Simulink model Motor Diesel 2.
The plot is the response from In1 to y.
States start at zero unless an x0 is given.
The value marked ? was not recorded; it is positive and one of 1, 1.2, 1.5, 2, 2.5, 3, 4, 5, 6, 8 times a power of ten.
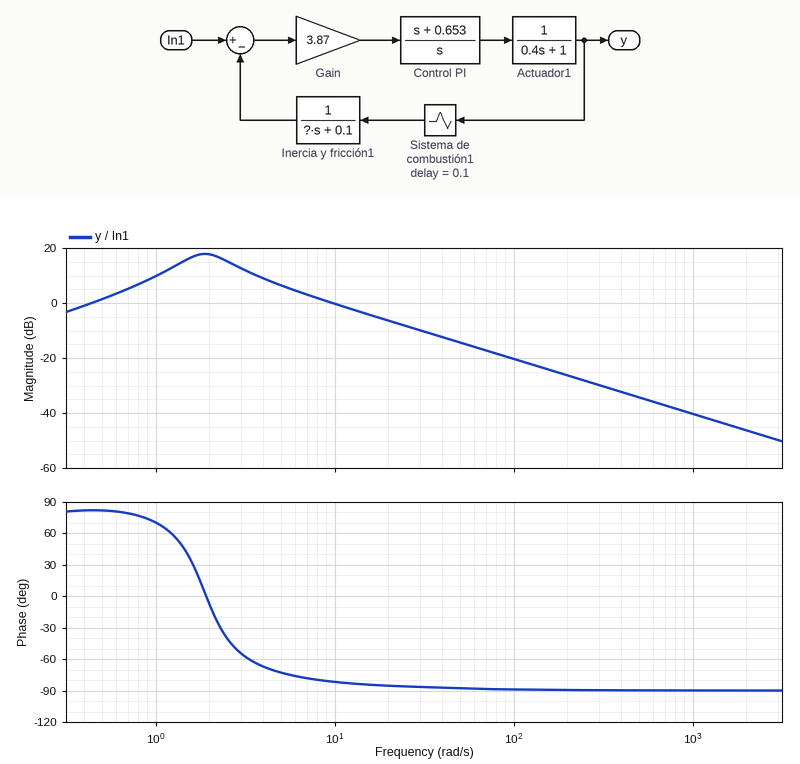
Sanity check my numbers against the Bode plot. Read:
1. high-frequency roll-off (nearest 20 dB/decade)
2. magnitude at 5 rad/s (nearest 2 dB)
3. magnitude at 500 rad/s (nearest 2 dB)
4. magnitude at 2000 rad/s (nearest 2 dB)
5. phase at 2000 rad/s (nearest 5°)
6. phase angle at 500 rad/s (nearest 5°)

-20 dB/decade
6 dB
-34 dB
-46 dB
-90°
-90°
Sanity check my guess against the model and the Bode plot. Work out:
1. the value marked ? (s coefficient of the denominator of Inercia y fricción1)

2
